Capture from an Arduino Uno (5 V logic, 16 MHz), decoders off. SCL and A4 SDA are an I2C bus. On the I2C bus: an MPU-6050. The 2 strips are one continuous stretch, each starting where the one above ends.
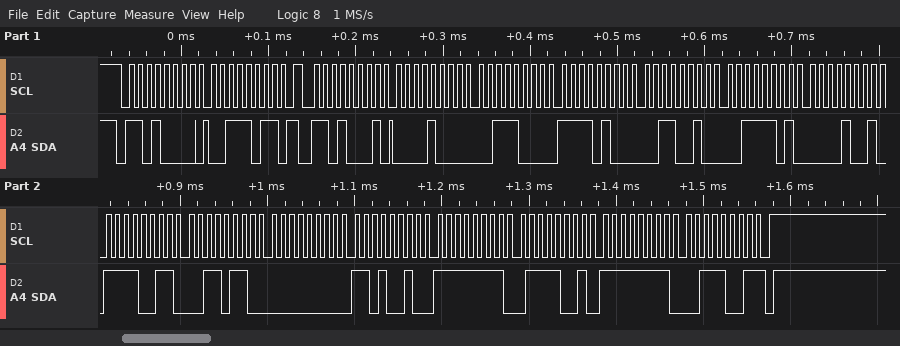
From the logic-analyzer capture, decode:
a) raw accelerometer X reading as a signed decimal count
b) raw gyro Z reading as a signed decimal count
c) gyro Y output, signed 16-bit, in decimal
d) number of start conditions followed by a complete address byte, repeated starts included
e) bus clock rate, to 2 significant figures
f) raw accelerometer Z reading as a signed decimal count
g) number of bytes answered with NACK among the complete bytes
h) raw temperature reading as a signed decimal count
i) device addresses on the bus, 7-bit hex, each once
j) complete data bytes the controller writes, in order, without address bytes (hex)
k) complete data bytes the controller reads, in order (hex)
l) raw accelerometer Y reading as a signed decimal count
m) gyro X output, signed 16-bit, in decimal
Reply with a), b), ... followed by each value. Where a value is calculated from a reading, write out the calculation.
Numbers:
a) 0x0838 = 2104
b) 0xFF39 = -199
c) 0xFF79 = -135
d) 2
e) 100 kHz
f) 0x3D09 = 15625
g) 1
h) 0xF336 = -3274
i) 0x68
j) 3B
k) 08 38 F4 32 3D 09 F3 36 00 D2 FF 79 FF 39
l) 0xF432 = -3022
m) 0x00D2 = 210
